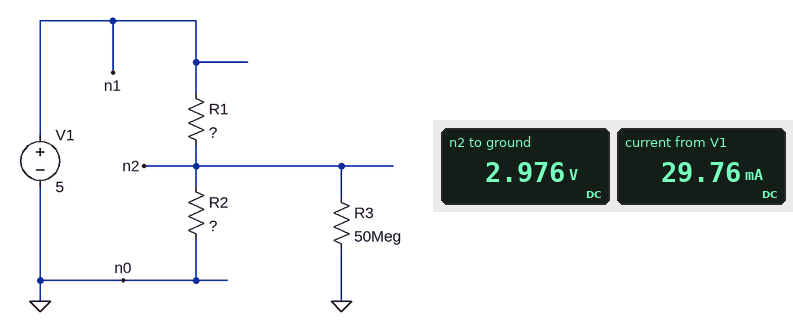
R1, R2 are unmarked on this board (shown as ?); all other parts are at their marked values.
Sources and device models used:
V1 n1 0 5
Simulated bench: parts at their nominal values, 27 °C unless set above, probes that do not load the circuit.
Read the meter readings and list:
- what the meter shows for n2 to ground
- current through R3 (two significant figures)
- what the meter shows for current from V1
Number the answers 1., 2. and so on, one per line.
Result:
1. 2.976 V
2. 60 nA
3. 29.76 mA
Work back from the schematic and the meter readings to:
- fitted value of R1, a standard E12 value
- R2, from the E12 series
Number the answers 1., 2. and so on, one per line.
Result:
1. 68 Ω
2. 100 Ω
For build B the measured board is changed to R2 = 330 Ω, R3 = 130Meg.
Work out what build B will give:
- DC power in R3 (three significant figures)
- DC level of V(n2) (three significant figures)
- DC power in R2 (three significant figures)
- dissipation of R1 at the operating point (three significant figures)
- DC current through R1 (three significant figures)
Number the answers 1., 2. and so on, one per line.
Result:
1. 132 nW
2. 4.15 V
3. 52.1 mW
4. 10.7 mW
5. 12.6 mA
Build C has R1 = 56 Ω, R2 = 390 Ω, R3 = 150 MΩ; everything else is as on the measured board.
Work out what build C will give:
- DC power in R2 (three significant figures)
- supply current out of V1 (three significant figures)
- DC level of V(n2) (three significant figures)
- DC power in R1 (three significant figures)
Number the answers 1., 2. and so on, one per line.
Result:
1. 49.0 mW
2. 11.2 mA
3. 4.37 V
4. 7.04 mW
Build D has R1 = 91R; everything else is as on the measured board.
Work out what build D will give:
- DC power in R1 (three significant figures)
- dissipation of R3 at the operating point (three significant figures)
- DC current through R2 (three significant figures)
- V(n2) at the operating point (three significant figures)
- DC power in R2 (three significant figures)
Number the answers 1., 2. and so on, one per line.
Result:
1. 62.4 mW
2. 137 nW
3. 26.2 mA
4. 2.62 V
5. 68.5 mW
